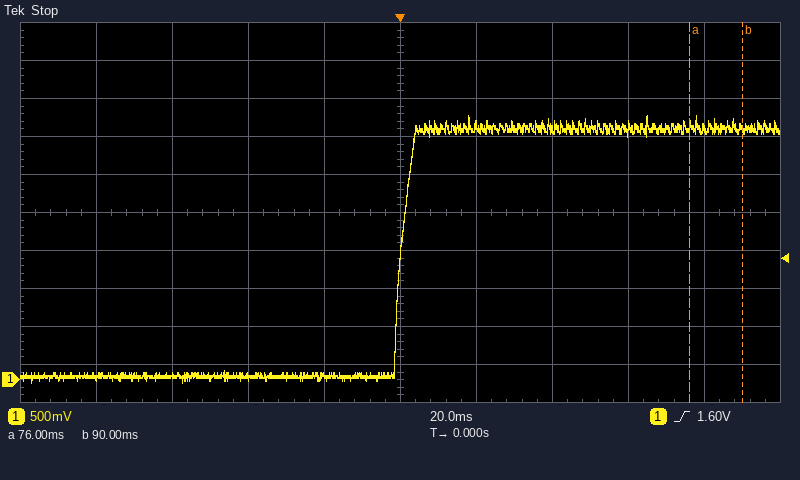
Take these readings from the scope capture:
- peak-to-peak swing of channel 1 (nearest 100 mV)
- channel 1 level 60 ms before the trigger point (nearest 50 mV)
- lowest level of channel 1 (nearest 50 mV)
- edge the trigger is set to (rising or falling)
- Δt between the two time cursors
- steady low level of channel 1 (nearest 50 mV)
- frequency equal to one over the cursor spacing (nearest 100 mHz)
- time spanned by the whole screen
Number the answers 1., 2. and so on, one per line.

1. 3.50 V
2. 50 mV
3. -50 mV
4. rising
5. 14 ms
6. 50 mV
7. 71.4 Hz
8. 200 ms
